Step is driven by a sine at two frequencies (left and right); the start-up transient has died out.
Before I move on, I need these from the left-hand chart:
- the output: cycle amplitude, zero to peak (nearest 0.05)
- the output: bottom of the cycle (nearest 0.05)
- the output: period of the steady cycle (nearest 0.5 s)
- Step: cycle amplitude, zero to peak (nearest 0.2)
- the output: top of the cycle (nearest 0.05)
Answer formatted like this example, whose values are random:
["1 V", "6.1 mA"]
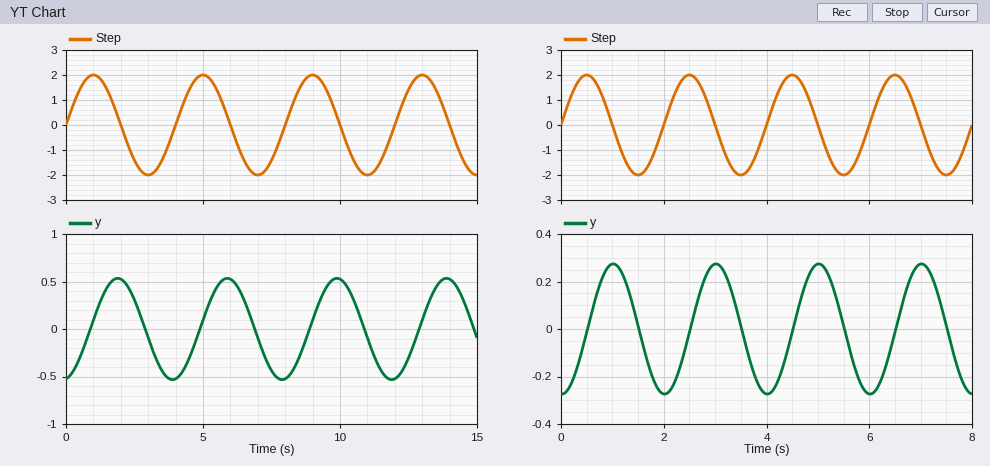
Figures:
["0.55", "-0.55", "4.0 s", "2.0", "0.55"]
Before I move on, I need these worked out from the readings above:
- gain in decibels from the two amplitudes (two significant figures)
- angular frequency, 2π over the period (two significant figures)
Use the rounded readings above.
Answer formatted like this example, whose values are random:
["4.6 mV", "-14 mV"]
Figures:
["-11 dB", "1.6 rad/s"]
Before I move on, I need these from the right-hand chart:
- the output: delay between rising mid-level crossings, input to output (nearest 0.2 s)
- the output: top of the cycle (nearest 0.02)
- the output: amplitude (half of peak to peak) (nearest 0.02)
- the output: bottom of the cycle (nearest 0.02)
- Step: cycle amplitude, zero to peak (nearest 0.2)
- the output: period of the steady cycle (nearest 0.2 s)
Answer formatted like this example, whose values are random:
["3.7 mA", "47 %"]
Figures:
["0.6 s", "0.28", "0.28", "-0.28", "2.0", "2.0 s"]
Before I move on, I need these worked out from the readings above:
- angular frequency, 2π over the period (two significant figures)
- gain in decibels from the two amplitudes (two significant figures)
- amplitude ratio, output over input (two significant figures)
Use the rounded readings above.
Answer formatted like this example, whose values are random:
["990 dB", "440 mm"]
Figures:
["3.1 rad/s", "-17 dB", "0.14"]
